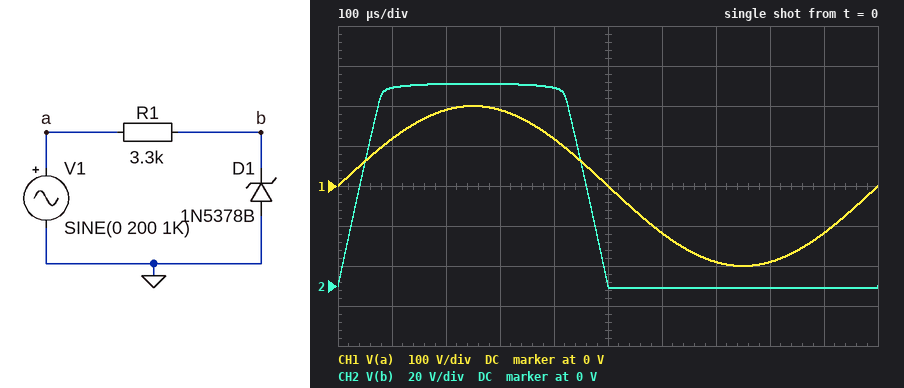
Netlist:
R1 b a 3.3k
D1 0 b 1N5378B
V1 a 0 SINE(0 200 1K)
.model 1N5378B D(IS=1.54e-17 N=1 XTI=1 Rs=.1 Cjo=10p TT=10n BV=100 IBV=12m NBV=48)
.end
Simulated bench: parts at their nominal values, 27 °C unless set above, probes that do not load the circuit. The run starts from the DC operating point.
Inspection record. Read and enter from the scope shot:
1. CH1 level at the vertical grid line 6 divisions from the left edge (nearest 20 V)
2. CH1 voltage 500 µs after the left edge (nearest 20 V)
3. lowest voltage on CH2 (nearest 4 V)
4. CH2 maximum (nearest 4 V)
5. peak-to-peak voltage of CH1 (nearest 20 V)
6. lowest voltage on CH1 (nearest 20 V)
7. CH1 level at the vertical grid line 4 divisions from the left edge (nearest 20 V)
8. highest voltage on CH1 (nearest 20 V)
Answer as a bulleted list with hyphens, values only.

- -120 V
- 0 V
- 0 V
- 100 V
- 400 V
- -200 V
- 120 V
- 200 V
